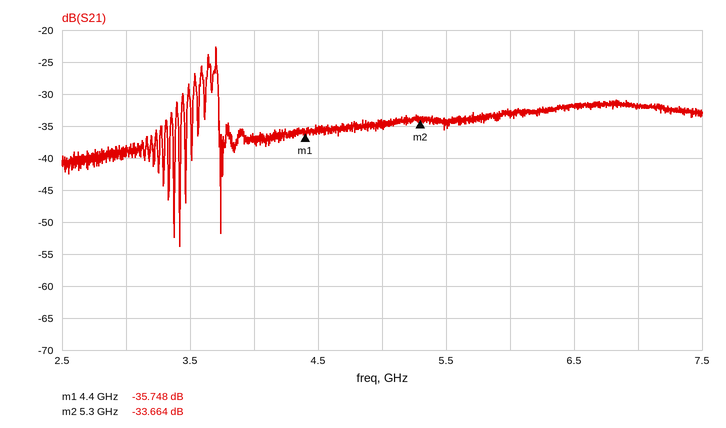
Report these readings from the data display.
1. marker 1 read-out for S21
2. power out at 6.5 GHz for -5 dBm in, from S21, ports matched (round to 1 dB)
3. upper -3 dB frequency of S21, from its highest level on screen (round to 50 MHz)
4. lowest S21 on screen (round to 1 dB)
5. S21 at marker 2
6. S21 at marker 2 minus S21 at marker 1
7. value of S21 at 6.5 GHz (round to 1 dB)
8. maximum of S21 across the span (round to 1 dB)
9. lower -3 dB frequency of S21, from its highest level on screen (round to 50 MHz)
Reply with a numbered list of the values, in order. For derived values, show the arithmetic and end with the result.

1. -35.748 dB
2. -5 dBm + (-32 dB) = -37 dBm
3. 3.70 GHz
4. -54 dB
5. -33.664 dB
6. -33.664 − (-35.748) = 2.084 dB
7. -32 dB
8. -23 dB
9. 3.70 GHz
